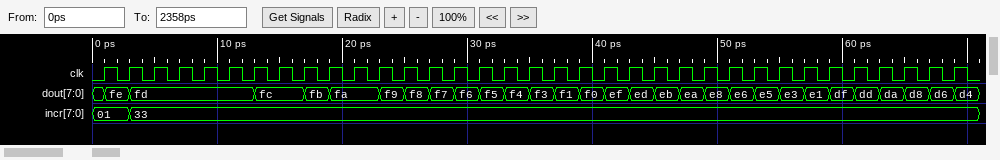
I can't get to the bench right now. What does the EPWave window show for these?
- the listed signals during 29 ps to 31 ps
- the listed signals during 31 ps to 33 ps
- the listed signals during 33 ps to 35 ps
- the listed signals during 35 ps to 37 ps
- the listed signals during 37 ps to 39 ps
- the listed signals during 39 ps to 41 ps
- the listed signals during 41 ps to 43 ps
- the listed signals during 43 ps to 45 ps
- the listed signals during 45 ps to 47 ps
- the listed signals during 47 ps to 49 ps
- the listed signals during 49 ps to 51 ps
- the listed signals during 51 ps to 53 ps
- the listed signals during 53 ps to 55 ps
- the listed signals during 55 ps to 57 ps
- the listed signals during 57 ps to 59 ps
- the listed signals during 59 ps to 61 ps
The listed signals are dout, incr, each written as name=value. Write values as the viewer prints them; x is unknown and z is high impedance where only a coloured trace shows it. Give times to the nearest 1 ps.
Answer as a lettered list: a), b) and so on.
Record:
a) dout=f6, incr=33
b) dout=f5, incr=33
c) dout=f4, incr=33
d) dout=f3, incr=33
e) dout=f1, incr=33
f) dout=f0, incr=33
g) dout=ef, incr=33
h) dout=ed, incr=33
i) dout=eb, incr=33
j) dout=ea, incr=33
k) dout=e8, incr=33
l) dout=e6, incr=33
m) dout=e5, incr=33
n) dout=e3, incr=33
o) dout=e1, incr=33
p) dout=df, incr=33
